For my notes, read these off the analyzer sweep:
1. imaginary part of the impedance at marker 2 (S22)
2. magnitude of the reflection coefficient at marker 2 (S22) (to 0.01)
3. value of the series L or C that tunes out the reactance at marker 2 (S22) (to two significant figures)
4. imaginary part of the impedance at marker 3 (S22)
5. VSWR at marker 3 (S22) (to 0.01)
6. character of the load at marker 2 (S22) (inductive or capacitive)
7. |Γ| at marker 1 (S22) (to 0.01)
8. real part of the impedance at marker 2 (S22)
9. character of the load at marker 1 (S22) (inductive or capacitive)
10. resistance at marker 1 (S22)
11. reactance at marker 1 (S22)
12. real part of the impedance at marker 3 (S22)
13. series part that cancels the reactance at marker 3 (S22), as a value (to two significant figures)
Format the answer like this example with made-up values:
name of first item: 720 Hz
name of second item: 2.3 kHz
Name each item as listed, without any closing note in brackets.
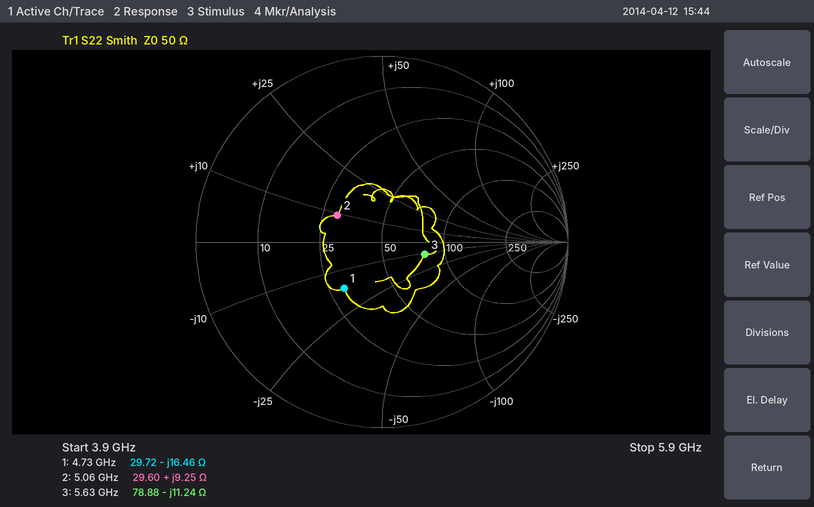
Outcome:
imaginary part of the impedance at marker 2: +9.25 Ω
magnitude of the reflection coefficient at marker 2 (S22): 0.28
value of the series L or C that tunes out the reactance at marker 2 (S22): 3.4 pF
imaginary part of the impedance at marker 3: -11.24 Ω
VSWR at marker 3 (S22): 1.63
character of the load at marker 2 (S22): inductive
|Γ| at marker 1 (S22): 0.32
real part of the impedance at marker 2: 29.60 Ω
character of the load at marker 1 (S22): capacitive
resistance at marker 1: 29.72 Ω
reactance at marker 1: -16.46 Ω
real part of the impedance at marker 3: 78.88 Ω
series part that cancels the reactance at marker 3 (S22), as a value: 320 pH
